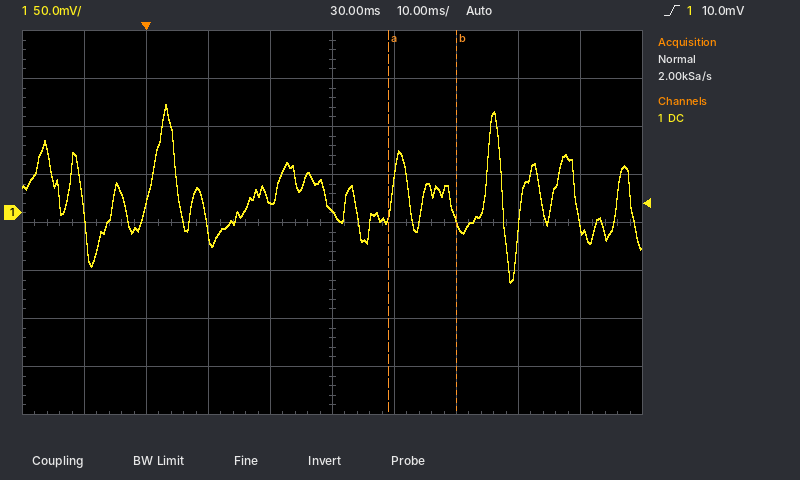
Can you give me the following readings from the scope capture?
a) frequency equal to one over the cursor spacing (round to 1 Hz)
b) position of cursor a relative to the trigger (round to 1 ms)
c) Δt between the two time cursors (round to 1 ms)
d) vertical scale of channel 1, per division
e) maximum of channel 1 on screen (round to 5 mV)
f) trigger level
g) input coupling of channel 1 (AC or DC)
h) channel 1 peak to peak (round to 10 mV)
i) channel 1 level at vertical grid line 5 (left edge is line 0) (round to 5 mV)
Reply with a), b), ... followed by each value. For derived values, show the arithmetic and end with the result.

a) 1 / 11 ms ≈ 91 Hz
b) +39 ms
c) 11 ms
d) 50 mV
e) 115 mV
f) 10.0 mV
g) DC
h) 190 mV
i) 0 mV
